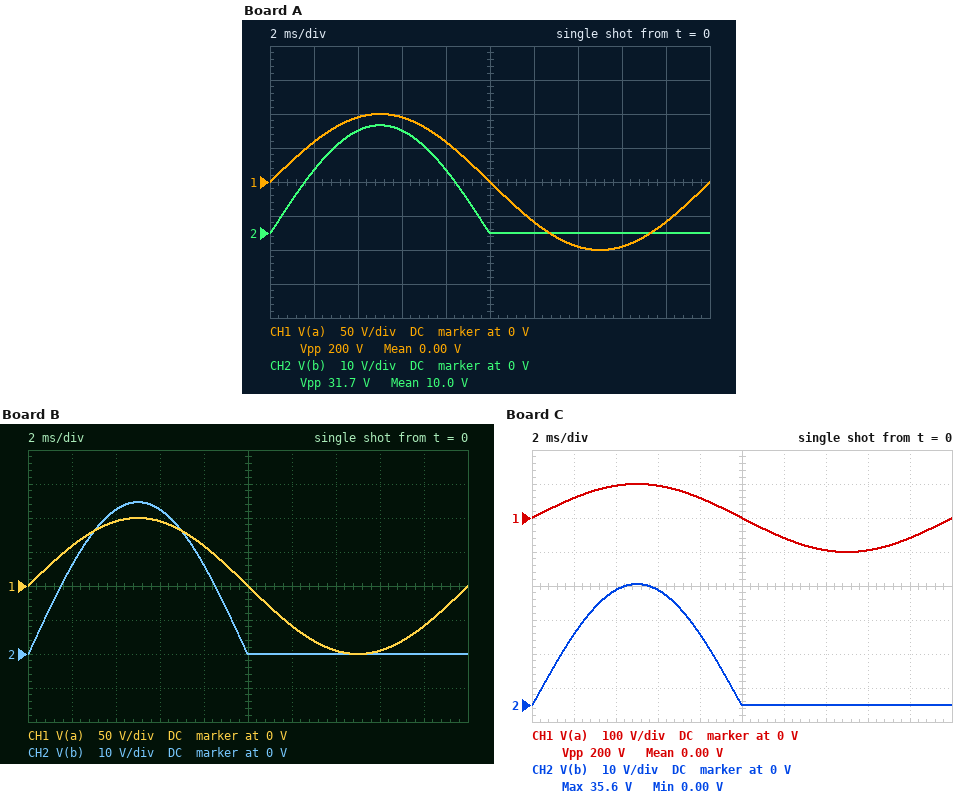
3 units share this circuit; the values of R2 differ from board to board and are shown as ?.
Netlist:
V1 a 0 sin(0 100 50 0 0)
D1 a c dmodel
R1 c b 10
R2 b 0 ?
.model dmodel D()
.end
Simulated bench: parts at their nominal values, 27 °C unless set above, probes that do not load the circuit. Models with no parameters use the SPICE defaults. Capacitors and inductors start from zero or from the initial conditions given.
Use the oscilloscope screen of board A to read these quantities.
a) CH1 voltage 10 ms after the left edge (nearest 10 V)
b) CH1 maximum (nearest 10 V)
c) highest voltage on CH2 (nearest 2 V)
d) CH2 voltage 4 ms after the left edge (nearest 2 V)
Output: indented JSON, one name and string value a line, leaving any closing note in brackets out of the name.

{
  "CH1 voltage 10 ms after the left edge": "0 V",
  "CH1 maximum": "100 V",
  "highest voltage on CH2": "32 V",
  "CH2 voltage 4 ms after the left edge": "30 V"
}
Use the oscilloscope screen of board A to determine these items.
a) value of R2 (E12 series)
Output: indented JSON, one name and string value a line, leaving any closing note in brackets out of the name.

{
  "value of R2": "4.7 Ω"
}
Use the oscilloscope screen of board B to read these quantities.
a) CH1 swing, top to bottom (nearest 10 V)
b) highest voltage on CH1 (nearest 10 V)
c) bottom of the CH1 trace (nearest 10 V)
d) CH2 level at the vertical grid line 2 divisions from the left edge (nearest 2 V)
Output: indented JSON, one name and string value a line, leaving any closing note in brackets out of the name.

{
  "CH1 swing, top to bottom": "200 V",
  "highest voltage on CH1": "100 V",
  "bottom of the CH1 trace": "-100 V",
  "CH2 level at the vertical grid line 2 divisions from the left edge": "42 V"
}
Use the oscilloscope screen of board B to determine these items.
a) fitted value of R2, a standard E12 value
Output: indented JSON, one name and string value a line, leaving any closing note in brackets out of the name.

{
  "fitted value of R2, a standard E12 value": "8.2 Ω"
}
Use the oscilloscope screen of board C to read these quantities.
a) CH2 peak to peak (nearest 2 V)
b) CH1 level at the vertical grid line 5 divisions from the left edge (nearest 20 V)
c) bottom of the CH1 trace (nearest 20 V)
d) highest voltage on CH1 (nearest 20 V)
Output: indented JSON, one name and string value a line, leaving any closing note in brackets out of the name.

{
  "CH2 peak to peak": "36 V",
  "CH1 level at the vertical grid line 5 divisions from the left edge": "0 V",
  "bottom of the CH1 trace": "-100 V",
  "highest voltage on CH1": "100 V"
}
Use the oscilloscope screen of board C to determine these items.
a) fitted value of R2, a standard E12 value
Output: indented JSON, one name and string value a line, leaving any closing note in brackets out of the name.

{
  "fitted value of R2, a standard E12 value": "5.6 Ω"
}
